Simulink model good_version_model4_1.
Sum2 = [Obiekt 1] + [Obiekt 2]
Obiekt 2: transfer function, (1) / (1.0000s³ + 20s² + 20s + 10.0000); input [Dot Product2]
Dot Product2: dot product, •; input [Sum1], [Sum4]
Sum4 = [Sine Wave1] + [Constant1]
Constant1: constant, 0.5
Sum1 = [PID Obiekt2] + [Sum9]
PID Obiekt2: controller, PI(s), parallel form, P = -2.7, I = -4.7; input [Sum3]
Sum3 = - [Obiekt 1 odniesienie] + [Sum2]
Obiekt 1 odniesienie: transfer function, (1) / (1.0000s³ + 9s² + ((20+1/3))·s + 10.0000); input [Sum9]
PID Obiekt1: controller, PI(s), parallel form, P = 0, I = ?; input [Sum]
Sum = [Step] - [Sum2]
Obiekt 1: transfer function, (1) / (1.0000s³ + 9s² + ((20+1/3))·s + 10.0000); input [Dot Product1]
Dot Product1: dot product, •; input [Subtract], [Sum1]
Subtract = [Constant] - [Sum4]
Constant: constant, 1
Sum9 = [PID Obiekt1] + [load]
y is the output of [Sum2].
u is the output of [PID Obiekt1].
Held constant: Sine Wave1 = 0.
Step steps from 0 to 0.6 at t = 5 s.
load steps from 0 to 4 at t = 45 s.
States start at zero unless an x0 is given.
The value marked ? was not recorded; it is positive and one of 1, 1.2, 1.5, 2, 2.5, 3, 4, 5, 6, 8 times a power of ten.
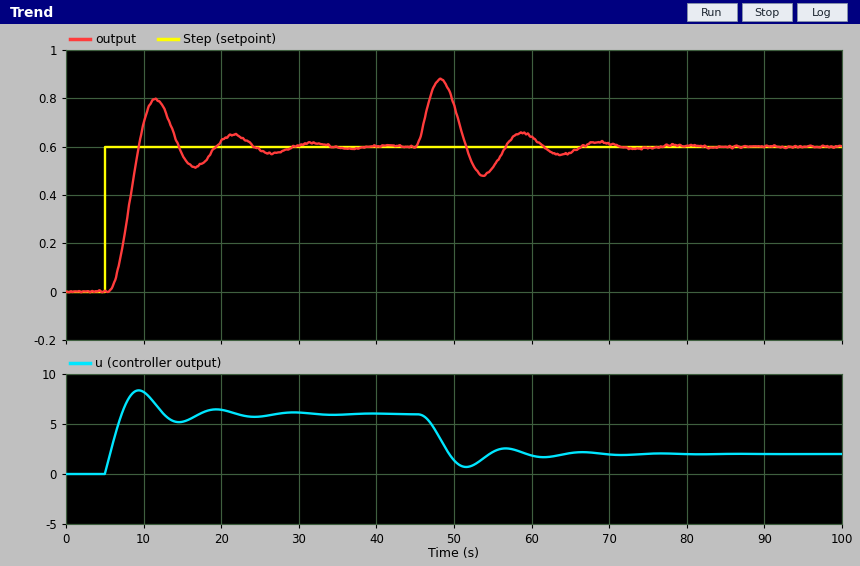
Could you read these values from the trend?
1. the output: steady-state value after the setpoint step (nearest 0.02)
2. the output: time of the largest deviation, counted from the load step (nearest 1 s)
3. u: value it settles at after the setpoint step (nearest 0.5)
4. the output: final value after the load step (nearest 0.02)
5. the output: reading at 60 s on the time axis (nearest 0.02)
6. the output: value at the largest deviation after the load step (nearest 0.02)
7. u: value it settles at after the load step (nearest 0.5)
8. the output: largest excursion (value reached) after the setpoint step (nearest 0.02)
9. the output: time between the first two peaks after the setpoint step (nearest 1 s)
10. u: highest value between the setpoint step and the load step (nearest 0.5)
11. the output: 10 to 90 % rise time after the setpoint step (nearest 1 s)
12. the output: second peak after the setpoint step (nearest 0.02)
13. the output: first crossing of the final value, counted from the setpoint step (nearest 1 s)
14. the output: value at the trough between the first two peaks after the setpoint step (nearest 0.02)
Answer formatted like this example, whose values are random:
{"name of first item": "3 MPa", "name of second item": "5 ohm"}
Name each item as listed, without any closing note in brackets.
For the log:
{"the output: steady-state value after the setpoint step": "0.60", "the output: time of the largest deviation, counted from the load step": "3 s", "u: value it settles at after the setpoint step": "6.0", "the output: final value after the load step": "0.60", "the output: reading at 60 s on the time axis": "0.64", "the output: value at the largest deviation after the load step": "0.88", "u: value it settles at after the load step": "2.0", "the output: largest excursion (value reached) after the setpoint step": "0.80", "the output: time between the first two peaks after the setpoint step": "10 s", "u: highest value between the setpoint step and the load step": "8.5", "the output: 10 to 90 % rise time after the setpoint step": "3 s", "the output: second peak after the setpoint step": "0.64", "the output: first crossing of the final value, counted from the setpoint step": "4 s", "the output: value at the trough between the first two peaks after the setpoint step": "0.52"}
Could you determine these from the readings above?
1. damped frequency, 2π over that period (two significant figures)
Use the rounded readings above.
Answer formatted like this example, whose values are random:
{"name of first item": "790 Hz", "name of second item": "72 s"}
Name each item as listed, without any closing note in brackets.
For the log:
{"damped frequency, 2π over that period": "0.63 rad/s"}
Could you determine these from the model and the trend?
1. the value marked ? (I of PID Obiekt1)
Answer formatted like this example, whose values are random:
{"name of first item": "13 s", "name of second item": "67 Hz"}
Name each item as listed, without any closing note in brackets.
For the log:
{"the value marked ?": "5"}
